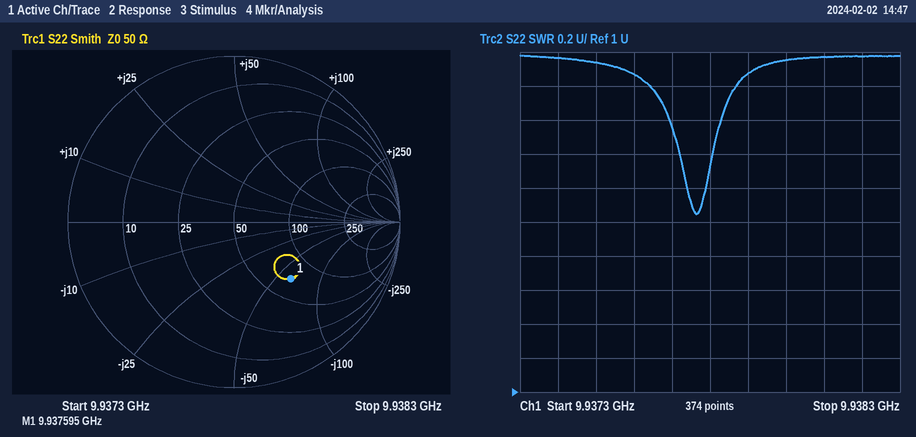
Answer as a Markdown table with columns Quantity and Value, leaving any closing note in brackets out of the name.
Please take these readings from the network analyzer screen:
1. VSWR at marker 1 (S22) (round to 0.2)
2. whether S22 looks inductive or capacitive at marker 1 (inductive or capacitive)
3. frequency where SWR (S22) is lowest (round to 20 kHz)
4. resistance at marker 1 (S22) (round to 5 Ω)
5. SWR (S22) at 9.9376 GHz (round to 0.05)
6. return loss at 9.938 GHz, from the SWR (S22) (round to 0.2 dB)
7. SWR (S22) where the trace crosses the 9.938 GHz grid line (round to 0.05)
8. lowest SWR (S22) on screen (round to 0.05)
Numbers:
| Quantity | Value |
|---|---|
| VSWR at marker 1 (S22) | 2.8 |
| whether S22 looks inductive or capacitive at marker 1 | capacitive |
| frequency where SWR (S22) is lowest | 9.93776 GHz |
| resistance at marker 1 (S22) | 70 Ω |
| SWR (S22) at 9.9376 GHz | 2.85 |
| return loss at 9.938 GHz, from the SWR (S22) | 6.2 dB |
| SWR (S22) where the trace crosses the 9.938 GHz grid line | 2.95 |
| lowest SWR (S22) on screen | 2.05 |
